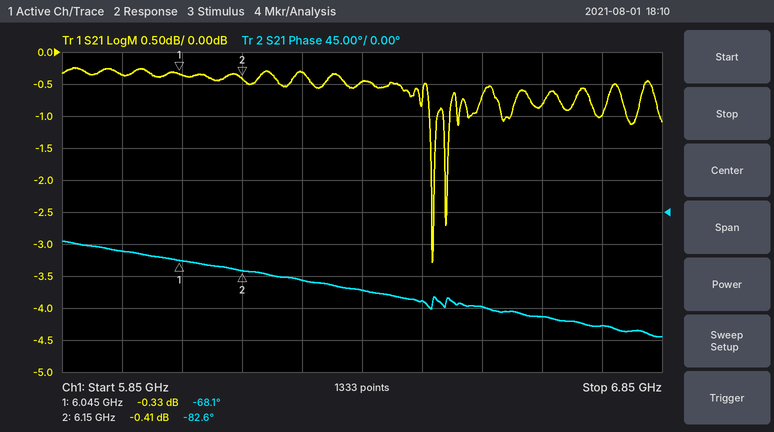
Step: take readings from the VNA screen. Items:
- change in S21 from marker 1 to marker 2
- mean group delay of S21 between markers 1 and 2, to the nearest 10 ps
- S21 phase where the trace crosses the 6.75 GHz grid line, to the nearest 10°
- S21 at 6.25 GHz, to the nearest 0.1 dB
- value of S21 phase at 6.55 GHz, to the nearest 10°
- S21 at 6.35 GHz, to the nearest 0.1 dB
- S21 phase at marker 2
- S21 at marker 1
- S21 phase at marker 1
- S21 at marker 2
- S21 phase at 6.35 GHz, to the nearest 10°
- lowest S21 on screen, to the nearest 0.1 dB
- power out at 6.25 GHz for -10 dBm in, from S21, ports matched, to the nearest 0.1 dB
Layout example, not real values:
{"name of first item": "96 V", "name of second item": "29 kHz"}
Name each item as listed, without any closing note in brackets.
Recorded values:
{"change in S21 from marker 1 to marker 2": "-0.08 dB", "mean group delay of S21 between markers 1 and 2, to the nearest 10 ps": "380 ps", "S21 phase where the trace crosses the 6.75 GHz grid line, to the nearest 10°": "-160°", "S21 at 6.25 GHz, to the nearest 0.1 dB": "-0.3 dB", "value of S21 phase at 6.55 GHz, to the nearest 10°": "-130°", "S21 at 6.35 GHz, to the nearest 0.1 dB": "-0.5 dB", "S21 phase at marker 2": "-82.6°", "S21 at marker 1": "-0.33 dB", "S21 phase at marker 1": "-68.1°", "S21 at marker 2": "-0.41 dB", "S21 phase at 6.35 GHz, to the nearest 10°": "-110°", "lowest S21 on screen, to the nearest 0.1 dB": "-3.3 dB", "power out at 6.25 GHz for -10 dBm in, from S21, ports matched, to the nearest 0.1 dB": "-10.3 dBm"}
